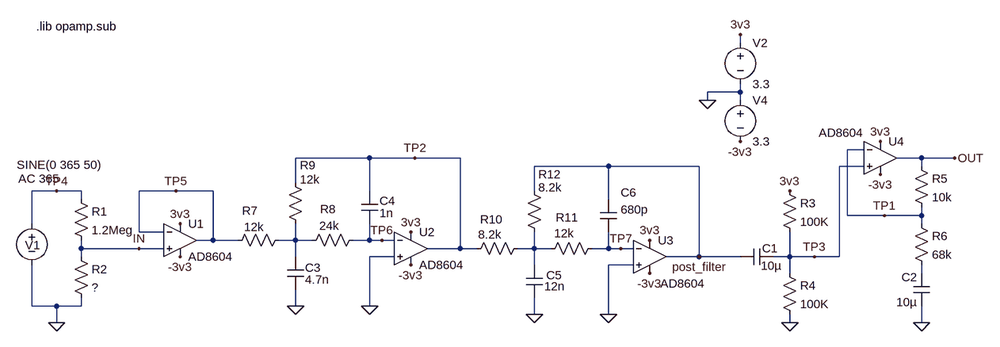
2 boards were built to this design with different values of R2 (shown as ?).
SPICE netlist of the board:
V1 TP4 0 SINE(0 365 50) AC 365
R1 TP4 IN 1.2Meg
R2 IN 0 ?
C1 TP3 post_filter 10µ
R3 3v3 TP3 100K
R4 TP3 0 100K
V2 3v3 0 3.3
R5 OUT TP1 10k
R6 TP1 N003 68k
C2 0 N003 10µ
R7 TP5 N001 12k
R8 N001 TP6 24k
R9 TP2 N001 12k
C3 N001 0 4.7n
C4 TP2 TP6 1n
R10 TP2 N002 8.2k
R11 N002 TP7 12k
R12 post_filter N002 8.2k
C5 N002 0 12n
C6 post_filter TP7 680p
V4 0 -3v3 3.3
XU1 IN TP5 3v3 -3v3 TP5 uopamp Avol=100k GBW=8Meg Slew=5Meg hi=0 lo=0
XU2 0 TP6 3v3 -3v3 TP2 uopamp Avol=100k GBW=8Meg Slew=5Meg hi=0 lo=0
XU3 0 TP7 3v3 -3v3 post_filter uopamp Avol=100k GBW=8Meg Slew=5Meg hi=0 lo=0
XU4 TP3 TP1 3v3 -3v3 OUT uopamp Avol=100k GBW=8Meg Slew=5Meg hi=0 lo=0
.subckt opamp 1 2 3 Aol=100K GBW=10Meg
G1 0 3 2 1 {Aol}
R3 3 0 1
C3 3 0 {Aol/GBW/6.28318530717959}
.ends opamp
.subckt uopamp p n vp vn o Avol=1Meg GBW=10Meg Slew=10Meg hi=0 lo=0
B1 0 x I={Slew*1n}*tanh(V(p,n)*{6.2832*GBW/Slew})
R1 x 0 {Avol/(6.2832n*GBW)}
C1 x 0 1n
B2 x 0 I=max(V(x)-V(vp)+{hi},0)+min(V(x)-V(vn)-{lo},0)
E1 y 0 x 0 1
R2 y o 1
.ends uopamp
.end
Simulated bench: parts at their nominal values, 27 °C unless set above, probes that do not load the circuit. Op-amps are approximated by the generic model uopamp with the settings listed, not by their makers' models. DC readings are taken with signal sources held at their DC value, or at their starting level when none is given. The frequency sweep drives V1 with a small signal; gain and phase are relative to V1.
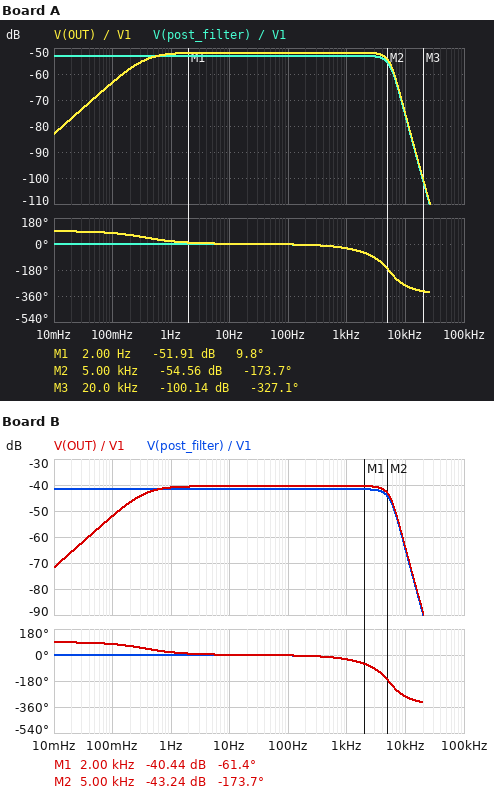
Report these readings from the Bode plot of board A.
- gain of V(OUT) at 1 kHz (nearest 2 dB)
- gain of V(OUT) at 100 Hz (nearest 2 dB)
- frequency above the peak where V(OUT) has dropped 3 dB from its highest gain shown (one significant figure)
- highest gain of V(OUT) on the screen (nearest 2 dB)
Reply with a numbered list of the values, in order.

1. -52 dB
2. -52 dB
3. 5 kHz
4. -52 dB
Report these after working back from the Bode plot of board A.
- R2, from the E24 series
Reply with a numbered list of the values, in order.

1. 2.7 kΩ
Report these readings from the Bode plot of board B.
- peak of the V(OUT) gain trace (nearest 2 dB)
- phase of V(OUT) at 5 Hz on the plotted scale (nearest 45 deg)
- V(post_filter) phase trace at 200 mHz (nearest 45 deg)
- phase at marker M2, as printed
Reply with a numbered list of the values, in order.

1. -40 dB
2. 0 deg
3. 0 deg
4. -173.7 deg
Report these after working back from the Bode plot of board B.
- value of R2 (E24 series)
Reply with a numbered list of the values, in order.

1. 10 kΩ
